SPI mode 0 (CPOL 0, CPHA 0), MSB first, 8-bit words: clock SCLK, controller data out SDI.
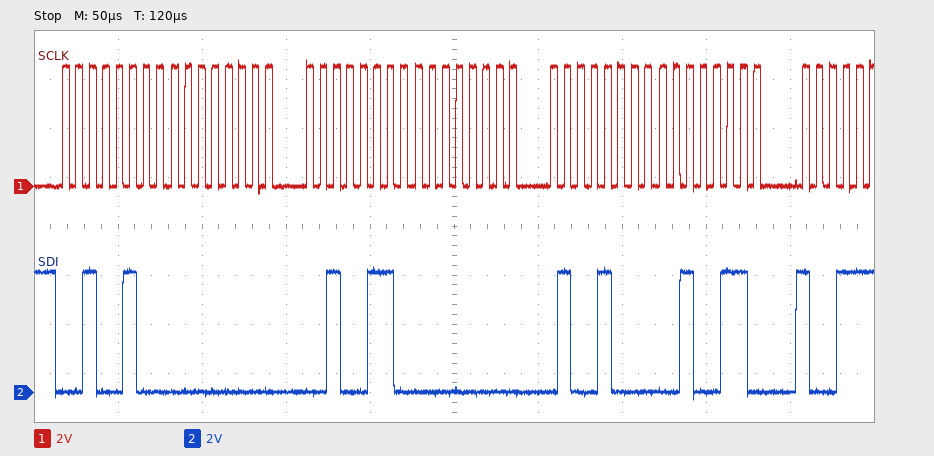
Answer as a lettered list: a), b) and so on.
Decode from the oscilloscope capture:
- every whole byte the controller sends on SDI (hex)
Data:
a) 24 00 26 00 48 26
